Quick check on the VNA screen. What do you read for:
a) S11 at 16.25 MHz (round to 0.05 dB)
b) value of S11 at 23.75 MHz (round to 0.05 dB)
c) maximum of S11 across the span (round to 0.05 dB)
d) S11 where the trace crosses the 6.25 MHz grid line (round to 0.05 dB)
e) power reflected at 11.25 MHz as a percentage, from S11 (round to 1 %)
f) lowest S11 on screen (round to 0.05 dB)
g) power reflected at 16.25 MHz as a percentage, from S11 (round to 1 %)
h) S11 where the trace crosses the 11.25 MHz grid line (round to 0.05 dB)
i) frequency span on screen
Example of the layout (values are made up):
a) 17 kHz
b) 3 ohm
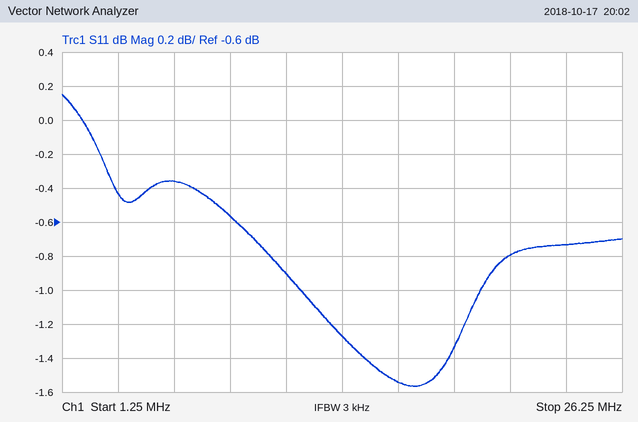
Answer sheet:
a) -1.55 dB
b) -0.75 dB
c) 0.15 dB
d) -0.35 dB
e) 81 %
f) -1.55 dB
g) 70 %
h) -0.90 dB
i) 25 MHz
